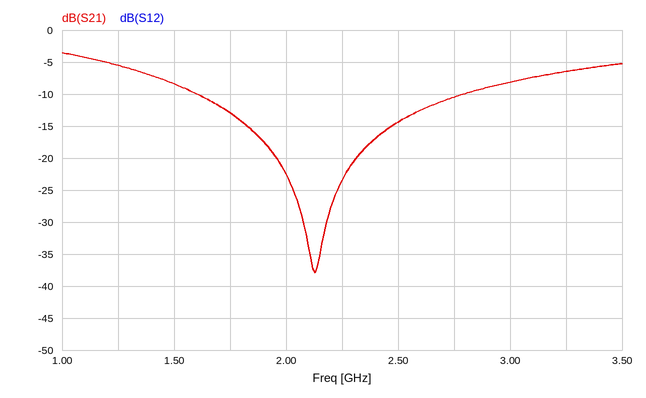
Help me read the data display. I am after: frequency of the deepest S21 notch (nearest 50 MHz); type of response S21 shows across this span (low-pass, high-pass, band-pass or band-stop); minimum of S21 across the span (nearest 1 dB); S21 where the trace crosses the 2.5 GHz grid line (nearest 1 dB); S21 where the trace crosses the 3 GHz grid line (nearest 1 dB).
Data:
2.15 GHz
band-stop
-38 dB
-14 dB
-8 dB
